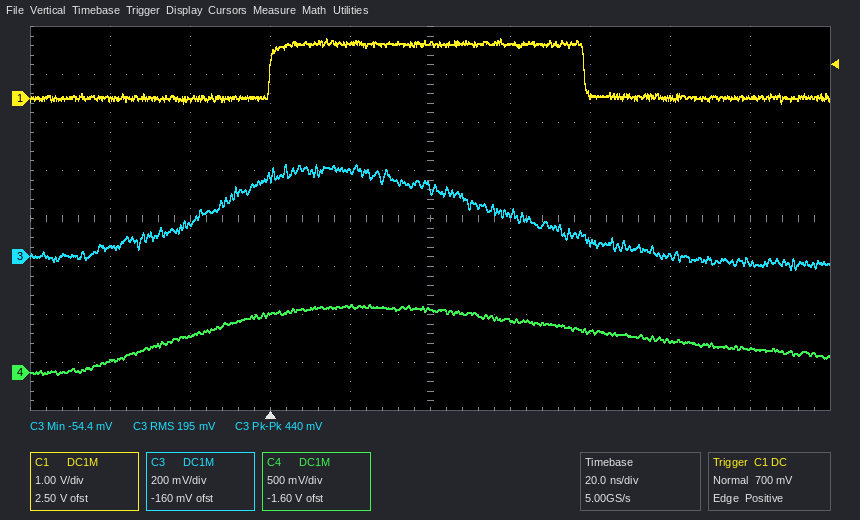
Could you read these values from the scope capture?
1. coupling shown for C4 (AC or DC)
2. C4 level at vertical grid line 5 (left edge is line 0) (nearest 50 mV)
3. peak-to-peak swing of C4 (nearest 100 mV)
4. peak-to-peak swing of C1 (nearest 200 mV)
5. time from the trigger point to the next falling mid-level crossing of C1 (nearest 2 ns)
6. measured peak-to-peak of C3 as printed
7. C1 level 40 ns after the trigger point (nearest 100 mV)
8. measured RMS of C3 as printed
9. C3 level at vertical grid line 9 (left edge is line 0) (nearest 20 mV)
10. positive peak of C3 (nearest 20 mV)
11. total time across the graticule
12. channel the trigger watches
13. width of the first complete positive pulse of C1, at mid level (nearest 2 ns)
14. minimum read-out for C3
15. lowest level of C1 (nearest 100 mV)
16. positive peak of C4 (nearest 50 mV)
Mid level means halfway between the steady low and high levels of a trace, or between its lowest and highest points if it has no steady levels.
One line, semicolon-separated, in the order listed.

DC; 650 mV; 700 mV; 1.4 V; 78 ns; 440 mV; 1.1 V; 195 mV; -20 mV; 380 mV; 200 ns; C1; 78 ns; -54.4 mV; -100 mV; 700 mV
